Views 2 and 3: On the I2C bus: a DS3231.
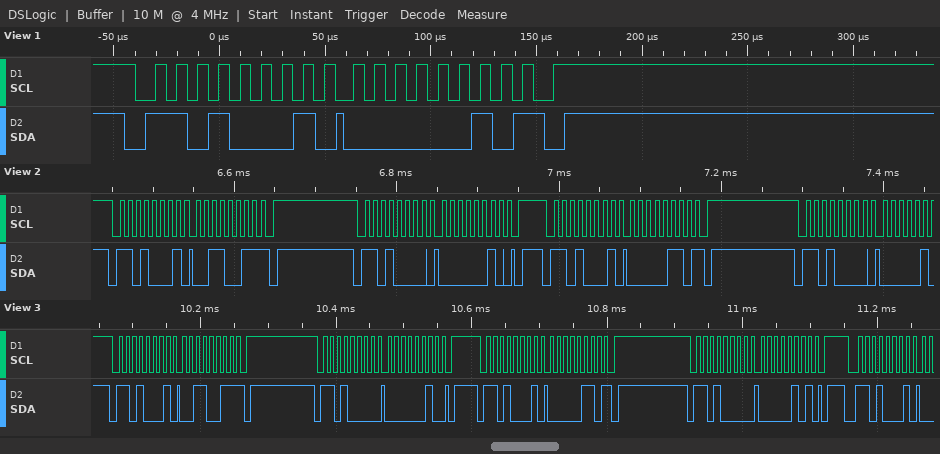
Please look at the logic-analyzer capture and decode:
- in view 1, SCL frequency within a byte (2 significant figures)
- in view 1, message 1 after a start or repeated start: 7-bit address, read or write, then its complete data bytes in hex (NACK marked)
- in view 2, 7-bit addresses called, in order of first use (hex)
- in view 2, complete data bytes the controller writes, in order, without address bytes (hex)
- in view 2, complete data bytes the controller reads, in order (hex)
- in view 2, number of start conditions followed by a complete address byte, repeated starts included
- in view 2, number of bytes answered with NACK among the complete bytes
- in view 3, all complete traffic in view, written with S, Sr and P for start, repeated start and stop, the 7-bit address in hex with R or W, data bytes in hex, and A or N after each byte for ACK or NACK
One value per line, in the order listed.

100 kHz
0x68 read: 02 NACK
0x68
02
33 06
4
2
S 68R A 33 N P S 68W A 02 A P S 68R A 06 N P S 68W A 05 A P S 68R A
